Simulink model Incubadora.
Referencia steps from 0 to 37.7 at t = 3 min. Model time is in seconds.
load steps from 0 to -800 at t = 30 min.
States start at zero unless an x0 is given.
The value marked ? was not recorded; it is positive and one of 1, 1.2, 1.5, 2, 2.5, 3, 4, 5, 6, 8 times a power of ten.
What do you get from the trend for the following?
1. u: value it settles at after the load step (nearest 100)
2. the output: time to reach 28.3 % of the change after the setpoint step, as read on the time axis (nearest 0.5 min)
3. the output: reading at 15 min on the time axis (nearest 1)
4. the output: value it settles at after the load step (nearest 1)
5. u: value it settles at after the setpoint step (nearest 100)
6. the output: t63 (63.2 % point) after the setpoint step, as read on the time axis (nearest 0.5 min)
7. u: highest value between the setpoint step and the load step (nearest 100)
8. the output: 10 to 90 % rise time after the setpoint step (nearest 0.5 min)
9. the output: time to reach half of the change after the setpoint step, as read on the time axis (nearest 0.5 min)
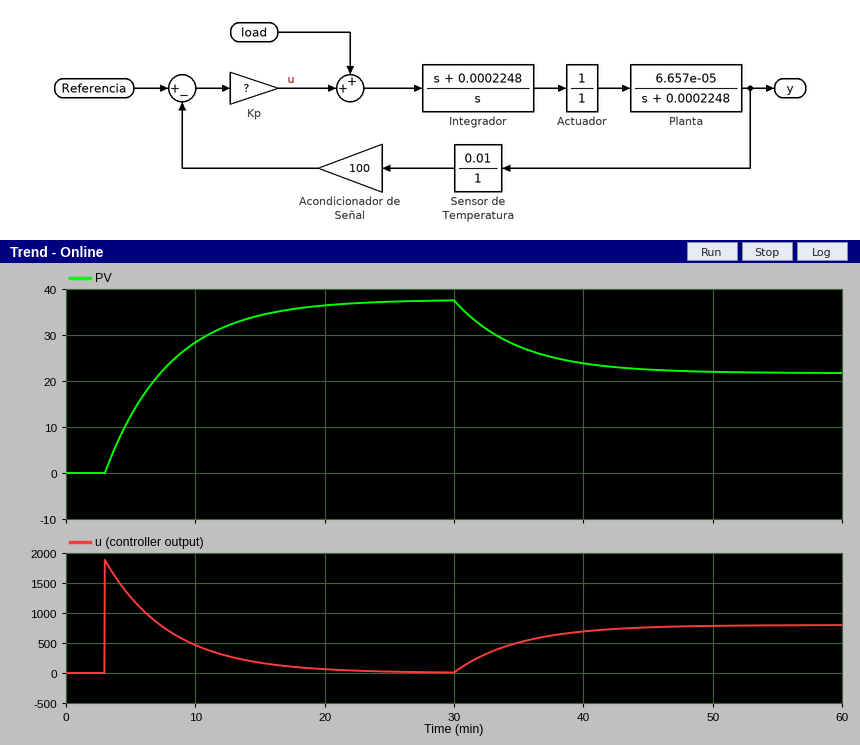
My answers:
800
4.5 min
34
22
0
8.0 min
1900
11.0 min
6.5 min
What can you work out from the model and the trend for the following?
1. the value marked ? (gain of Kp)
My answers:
50
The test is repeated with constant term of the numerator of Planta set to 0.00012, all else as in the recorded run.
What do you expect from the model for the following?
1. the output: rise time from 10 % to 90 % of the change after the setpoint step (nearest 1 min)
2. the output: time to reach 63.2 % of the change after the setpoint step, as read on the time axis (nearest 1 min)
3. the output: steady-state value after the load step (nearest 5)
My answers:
6 min
6 min
20
